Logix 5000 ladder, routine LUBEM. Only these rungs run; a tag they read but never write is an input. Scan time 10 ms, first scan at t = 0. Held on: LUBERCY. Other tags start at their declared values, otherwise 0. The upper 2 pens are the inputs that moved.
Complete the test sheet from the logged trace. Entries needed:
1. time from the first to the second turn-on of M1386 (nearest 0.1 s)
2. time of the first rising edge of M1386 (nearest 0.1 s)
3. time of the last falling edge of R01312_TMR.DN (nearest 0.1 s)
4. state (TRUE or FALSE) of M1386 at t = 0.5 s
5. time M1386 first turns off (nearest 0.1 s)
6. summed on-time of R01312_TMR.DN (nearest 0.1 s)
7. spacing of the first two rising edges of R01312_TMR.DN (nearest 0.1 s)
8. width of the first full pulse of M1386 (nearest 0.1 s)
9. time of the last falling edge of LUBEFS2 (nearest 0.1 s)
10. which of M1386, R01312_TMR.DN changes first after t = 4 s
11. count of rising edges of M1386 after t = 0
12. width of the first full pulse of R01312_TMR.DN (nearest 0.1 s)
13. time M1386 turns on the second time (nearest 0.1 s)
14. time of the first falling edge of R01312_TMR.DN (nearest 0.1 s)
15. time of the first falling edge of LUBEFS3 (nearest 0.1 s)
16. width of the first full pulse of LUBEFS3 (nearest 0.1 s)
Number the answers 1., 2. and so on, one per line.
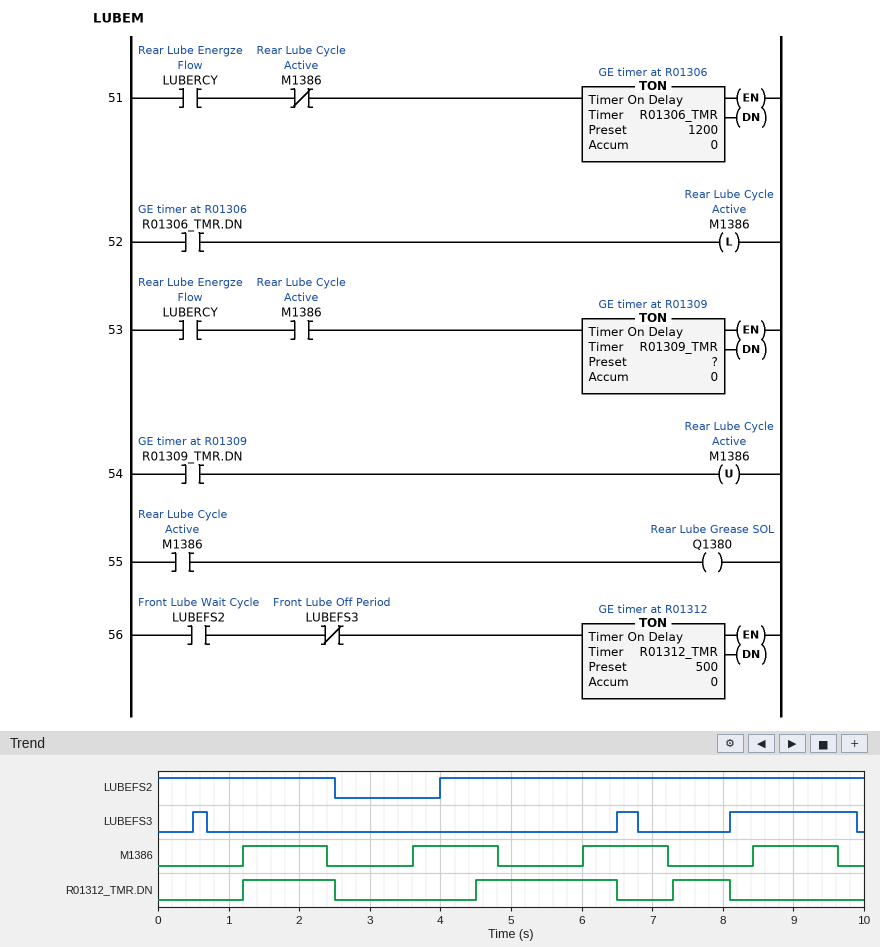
1. 2.4 s
2. 1.2 s
3. 8.1 s
4. FALSE
5. 2.4 s
6. 4.1 s
7. 3.3 s
8. 1.2 s
9. 2.5 s
10. R01312_TMR.DN
11. 4
12. 1.3 s
13. 3.6 s
14. 2.5 s
15. 0.7 s
16. 0.2 s
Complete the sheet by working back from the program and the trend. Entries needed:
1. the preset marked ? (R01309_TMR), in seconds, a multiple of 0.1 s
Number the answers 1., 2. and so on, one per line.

1. 1.2 s
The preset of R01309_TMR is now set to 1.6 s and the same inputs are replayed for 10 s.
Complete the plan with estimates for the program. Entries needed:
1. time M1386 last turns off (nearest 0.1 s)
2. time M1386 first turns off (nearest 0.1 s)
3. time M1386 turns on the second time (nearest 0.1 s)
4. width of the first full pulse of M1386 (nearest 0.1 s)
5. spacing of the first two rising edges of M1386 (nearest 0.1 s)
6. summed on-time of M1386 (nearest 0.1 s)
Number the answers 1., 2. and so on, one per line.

1. 8.4 s
2. 2.8 s
3. 4.0 s
4. 1.6 s
5. 2.8 s
6. 5.2 s
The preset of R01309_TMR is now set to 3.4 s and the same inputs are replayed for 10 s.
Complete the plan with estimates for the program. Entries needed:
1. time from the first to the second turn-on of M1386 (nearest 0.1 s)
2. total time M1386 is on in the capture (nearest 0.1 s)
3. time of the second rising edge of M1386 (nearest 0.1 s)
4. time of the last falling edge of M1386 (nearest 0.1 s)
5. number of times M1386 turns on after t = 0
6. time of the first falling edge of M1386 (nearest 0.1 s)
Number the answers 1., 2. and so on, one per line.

1. 4.6 s
2. 6.8 s
3. 5.8 s
4. 9.2 s
5. 2
6. 4.6 s
